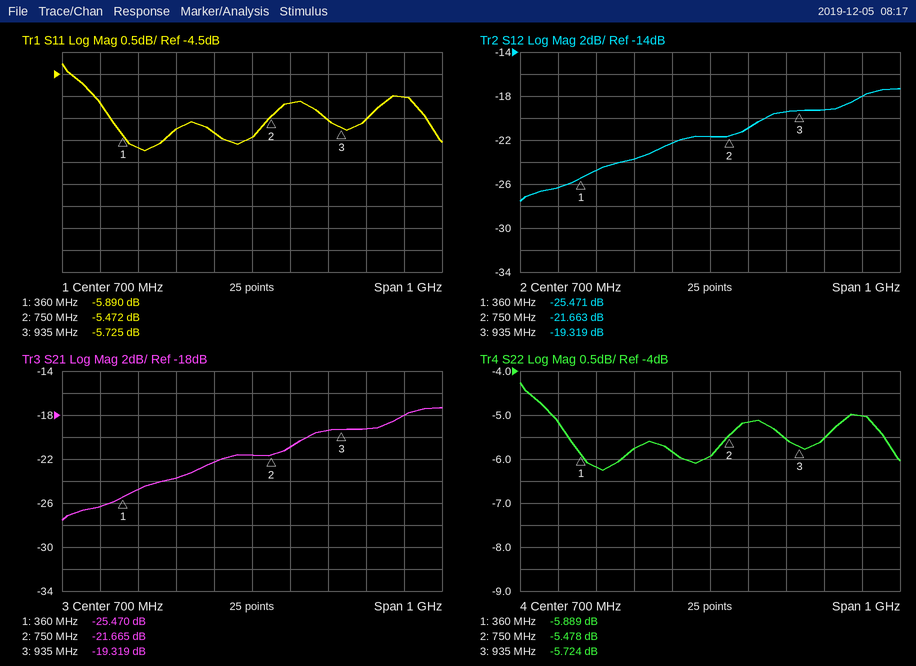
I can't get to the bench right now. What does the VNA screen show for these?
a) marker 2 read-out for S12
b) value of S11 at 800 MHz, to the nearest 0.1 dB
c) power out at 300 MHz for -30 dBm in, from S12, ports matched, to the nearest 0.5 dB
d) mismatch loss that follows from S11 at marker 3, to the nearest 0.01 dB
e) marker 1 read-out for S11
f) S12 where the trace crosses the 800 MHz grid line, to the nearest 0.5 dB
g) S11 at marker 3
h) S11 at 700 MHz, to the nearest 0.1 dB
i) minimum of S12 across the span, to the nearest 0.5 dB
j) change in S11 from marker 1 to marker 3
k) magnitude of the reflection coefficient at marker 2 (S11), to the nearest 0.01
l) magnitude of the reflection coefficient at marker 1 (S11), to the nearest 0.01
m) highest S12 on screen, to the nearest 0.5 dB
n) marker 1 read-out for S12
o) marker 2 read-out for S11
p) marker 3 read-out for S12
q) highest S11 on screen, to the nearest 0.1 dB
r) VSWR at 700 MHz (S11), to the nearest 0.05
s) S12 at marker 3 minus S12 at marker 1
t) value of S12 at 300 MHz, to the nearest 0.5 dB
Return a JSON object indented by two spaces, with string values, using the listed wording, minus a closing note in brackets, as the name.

{
  "marker 2 read-out for S12": "-21.663 dB",
  "value of S11 at 800 MHz, to the nearest 0.1 dB": "-5.2 dB",
  "power out at 300 MHz for -30 dBm in, from S12, ports matched, to the nearest 0.5 dB": "-56.5 dBm",
  "mismatch loss that follows from S11 at marker 3, to the nearest 0.01 dB": "1.35 dB",
  "marker 1 read-out for S11": "-5.890 dB",
  "S12 where the trace crosses the 800 MHz grid line, to the nearest 0.5 dB": "-21.0 dB",
  "S11 at marker 3": "-5.725 dB",
  "S11 at 700 MHz, to the nearest 0.1 dB": "-5.9 dB",
  "minimum of S12 across the span, to the nearest 0.5 dB": "-27.5 dB",
  "change in S11 from marker 1 to marker 3": "0.165 dB",
  "magnitude of the reflection coefficient at marker 2 (S11), to the nearest 0.01": "0.53",
  "magnitude of the reflection coefficient at marker 1 (S11), to the nearest 0.01": "0.51",
  "highest S12 on screen, to the nearest 0.5 dB": "-17.5 dB",
  "marker 1 read-out for S12": "-25.471 dB",
  "marker 2 read-out for S11": "-5.472 dB",
  "marker 3 read-out for S12": "-19.319 dB",
  "highest S11 on screen, to the nearest 0.1 dB": "-4.3 dB",
  "VSWR at 700 MHz (S11), to the nearest 0.05": "3.05",
  "S12 at marker 3 minus S12 at marker 1": "6.152 dB",
  "value of S12 at 300 MHz, to the nearest 0.5 dB": "-26.5 dB"
}
